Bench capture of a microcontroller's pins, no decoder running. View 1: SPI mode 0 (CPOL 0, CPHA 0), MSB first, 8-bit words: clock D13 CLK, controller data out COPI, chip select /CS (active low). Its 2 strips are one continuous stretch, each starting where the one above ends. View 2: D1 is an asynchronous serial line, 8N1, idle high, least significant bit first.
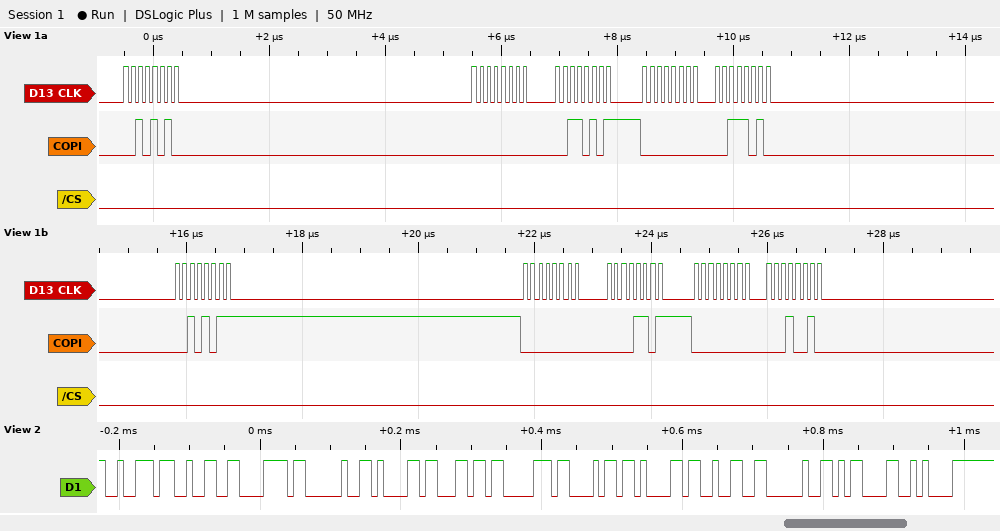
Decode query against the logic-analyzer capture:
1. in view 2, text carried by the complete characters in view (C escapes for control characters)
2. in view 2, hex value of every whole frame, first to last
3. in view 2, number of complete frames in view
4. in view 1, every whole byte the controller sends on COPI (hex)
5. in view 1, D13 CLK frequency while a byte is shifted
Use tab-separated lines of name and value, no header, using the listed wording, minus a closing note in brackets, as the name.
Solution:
in view 2, text carried by the complete characters in view	"r2x alpha2 \r\n"
in view 2, hex value of every whole frame, first to last	72 32 78 20 61 6C 70 68 61 32 20 0D 0A
in view 2, number of complete frames in view	13
in view 1, every whole byte the controller sends on COPI	2A 00 35 00 3A 2B 00 0D 00 12
in view 1, D13 CLK frequency while a byte is shifted	8 MHz
